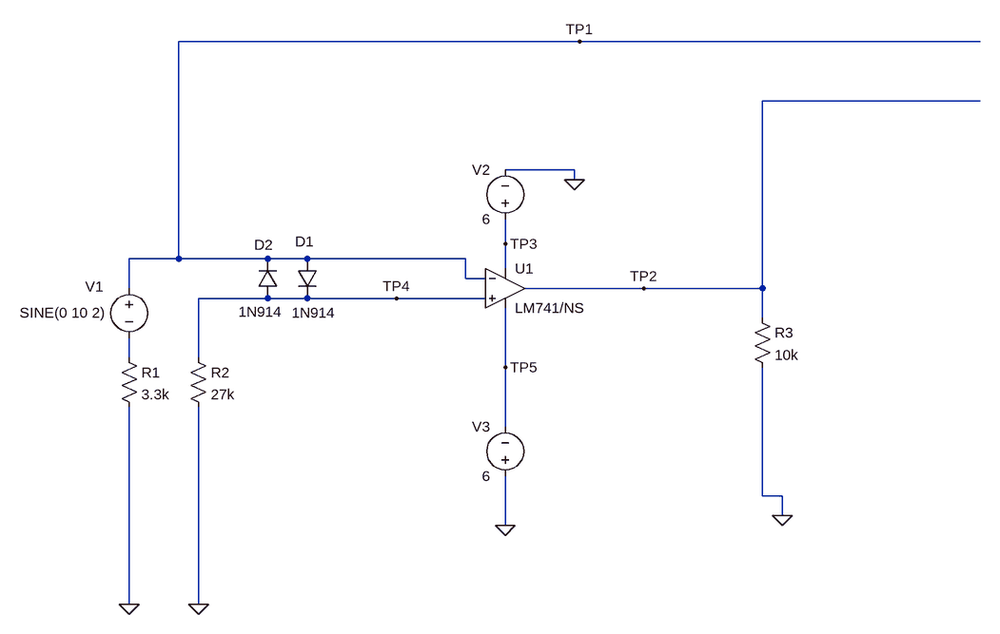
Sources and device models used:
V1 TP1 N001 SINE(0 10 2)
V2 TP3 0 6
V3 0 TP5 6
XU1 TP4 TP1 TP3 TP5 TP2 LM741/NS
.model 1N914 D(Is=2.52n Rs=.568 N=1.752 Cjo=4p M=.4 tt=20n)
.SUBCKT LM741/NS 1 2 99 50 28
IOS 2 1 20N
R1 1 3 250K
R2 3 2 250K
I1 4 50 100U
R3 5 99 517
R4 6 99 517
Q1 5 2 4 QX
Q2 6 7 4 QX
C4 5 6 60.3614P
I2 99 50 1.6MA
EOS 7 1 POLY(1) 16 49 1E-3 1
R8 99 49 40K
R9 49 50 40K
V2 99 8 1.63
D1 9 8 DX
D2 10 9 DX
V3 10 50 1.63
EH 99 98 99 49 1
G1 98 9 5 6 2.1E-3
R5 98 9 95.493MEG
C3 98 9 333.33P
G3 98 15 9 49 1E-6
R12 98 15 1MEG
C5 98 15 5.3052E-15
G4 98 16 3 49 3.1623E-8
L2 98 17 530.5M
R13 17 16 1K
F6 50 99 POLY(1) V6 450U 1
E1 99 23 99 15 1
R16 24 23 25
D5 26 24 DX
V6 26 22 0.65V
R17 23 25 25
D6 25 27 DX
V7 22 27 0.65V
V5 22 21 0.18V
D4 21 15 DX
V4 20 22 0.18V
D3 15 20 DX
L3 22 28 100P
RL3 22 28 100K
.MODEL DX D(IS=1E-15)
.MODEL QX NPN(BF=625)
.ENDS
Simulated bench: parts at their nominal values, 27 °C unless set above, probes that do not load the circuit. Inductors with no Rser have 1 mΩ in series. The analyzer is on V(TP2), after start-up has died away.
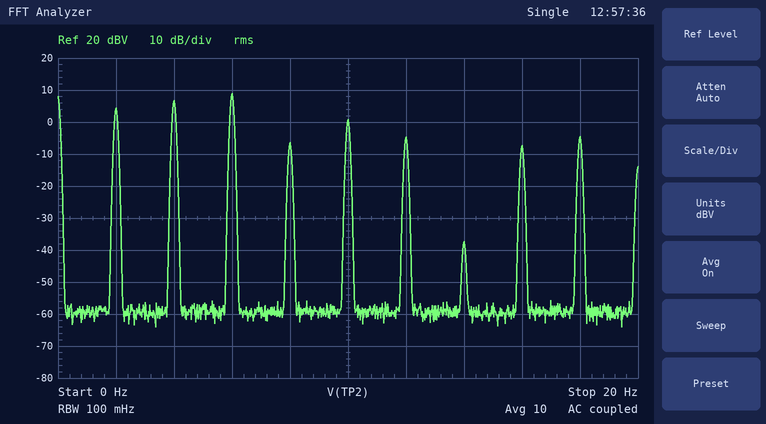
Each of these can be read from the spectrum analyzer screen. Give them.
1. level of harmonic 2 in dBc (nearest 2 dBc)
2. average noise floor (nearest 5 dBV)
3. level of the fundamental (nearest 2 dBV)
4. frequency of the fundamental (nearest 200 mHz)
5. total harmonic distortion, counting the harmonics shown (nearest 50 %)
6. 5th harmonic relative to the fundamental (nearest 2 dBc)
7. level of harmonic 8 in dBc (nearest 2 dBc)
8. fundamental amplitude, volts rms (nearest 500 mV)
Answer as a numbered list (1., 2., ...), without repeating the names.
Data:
1. 2 dBc
2. -60 dBV
3. 4 dBV
4. 2.0 Hz
5. 250 %
6. -4 dBc
7. -12 dBc
8. 1.5 V
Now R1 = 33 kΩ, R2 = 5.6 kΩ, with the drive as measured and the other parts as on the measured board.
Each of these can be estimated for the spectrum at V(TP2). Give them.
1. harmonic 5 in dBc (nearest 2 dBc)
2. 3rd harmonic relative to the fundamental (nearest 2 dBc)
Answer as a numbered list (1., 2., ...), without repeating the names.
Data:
1. -14 dBc
2. -10 dBc
